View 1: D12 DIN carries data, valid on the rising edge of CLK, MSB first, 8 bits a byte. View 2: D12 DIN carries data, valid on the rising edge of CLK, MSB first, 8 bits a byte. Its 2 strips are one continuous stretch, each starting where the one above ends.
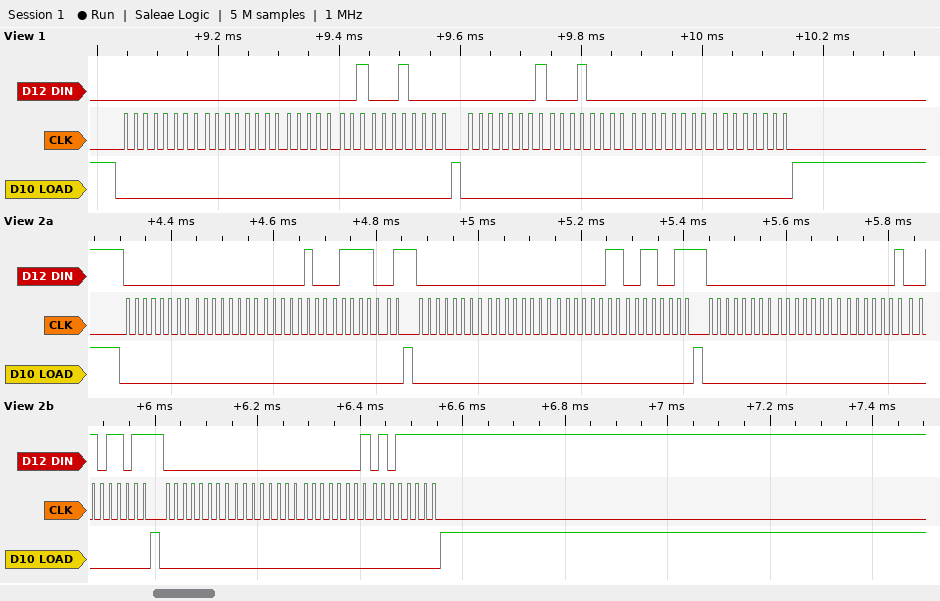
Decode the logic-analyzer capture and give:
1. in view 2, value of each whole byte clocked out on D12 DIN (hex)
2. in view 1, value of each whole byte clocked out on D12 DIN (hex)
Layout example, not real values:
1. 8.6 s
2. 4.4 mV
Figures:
1. 00 00 04 79 00 00 03 33 00 00 02 5B 00 00 01 5F
2. 00 00 01 10 01 10 00 00
